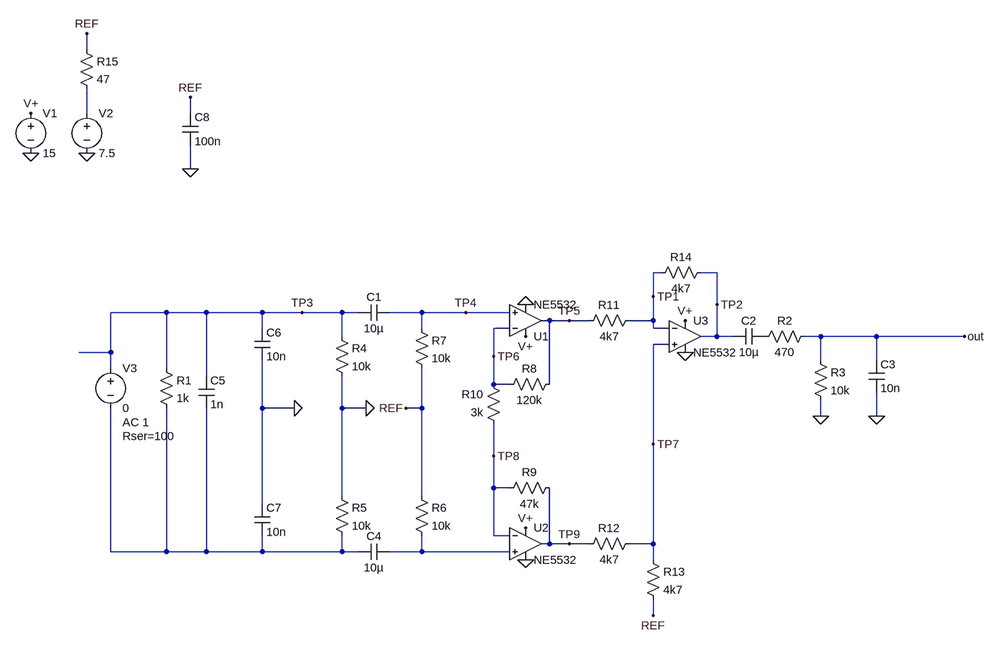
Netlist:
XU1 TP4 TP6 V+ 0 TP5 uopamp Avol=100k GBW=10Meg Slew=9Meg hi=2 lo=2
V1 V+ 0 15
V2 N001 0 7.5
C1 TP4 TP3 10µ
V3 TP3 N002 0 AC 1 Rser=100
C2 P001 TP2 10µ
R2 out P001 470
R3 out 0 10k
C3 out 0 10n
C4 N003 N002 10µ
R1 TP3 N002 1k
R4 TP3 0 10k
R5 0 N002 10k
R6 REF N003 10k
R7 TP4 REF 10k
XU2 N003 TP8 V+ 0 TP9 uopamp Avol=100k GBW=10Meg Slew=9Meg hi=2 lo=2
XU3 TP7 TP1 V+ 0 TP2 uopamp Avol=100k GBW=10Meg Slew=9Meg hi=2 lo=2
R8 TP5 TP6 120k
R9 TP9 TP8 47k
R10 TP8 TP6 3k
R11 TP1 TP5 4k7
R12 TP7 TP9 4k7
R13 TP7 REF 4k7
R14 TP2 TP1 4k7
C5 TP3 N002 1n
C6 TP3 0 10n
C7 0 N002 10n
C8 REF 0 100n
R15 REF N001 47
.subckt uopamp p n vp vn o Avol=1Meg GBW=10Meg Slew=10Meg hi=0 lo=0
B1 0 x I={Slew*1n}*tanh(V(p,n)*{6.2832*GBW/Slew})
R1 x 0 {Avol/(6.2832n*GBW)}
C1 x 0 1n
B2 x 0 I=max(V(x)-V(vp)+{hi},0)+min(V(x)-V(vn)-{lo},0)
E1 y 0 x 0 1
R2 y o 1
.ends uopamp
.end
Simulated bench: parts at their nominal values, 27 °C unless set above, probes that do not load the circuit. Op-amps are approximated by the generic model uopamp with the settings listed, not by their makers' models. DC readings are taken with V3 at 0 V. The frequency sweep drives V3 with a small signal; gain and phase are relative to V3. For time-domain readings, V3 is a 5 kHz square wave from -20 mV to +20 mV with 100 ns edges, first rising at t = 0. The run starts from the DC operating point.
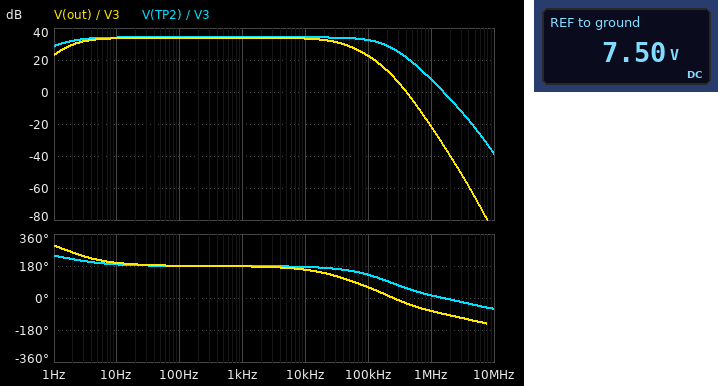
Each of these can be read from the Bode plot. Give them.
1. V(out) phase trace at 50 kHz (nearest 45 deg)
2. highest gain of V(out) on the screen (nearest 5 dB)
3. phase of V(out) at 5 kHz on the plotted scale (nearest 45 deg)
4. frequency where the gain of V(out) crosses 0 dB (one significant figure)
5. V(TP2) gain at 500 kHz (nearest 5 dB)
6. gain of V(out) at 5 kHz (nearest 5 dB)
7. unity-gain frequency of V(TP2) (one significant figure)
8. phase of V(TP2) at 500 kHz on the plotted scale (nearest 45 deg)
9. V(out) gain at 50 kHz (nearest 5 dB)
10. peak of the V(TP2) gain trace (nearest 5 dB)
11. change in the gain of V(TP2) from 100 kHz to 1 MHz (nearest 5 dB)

90 deg
35 dB
180 deg
400 kHz
20 dB
35 dB
2 MHz
45 deg
30 dB
35 dB
-25 dB
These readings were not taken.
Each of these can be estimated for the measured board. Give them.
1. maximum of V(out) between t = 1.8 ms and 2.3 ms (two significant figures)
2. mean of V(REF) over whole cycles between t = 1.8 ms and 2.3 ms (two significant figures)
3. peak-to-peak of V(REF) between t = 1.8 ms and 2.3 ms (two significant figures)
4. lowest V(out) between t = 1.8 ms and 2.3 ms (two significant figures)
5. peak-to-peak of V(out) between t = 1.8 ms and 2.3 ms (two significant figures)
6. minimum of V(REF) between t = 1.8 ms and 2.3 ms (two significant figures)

41 mV
7.5 V
2.9 mV
-1.9 V
2.0 V
7.5 V
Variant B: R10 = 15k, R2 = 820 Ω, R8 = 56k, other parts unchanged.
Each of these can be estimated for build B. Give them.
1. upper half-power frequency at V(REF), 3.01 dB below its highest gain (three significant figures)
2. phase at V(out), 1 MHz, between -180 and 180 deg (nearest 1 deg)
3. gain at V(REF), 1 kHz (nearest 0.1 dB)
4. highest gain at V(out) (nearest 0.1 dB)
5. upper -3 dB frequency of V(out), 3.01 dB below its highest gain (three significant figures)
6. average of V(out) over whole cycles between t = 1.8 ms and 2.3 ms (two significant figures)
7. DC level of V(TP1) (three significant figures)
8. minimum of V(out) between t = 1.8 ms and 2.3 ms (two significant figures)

33.4 kHz
-32 deg
-35.8 dB
16.3 dB
20.9 kHz
-130 mV
7.50 V
-260 mV
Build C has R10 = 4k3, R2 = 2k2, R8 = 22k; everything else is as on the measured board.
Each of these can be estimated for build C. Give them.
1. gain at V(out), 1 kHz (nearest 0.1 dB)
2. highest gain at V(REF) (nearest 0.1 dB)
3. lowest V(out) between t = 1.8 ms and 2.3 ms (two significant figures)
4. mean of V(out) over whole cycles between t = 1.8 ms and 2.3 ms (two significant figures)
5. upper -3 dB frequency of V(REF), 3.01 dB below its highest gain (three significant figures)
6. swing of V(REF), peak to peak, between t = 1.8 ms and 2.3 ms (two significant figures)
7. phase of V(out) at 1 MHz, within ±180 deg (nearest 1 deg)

22.0 dB
-25.8 dB
-490 mV
-240 mV
33.3 kHz
2.0 mV
-54 deg
